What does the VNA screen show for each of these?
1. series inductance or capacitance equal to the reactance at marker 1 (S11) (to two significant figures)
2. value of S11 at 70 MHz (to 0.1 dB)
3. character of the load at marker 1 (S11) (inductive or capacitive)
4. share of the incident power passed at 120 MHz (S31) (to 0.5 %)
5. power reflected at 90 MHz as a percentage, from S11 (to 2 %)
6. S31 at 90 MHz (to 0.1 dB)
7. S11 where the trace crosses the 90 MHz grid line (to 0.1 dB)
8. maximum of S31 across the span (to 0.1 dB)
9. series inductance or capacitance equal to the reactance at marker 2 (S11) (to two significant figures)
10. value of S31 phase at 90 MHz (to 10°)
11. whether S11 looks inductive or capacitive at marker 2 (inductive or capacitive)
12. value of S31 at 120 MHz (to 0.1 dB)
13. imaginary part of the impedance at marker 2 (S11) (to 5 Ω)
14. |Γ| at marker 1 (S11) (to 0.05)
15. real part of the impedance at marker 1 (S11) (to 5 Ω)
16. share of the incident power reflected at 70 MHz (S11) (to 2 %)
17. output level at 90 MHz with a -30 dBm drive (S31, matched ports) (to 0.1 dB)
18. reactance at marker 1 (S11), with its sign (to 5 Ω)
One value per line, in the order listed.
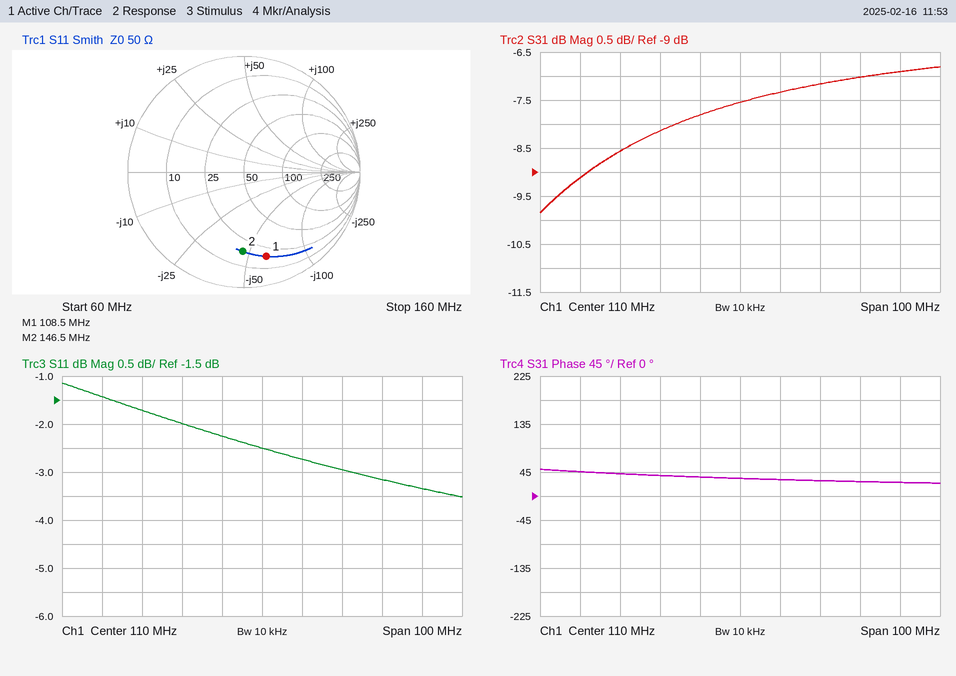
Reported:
24 pF
-1.4 dB
capacitive
18.5 %
64 %
-8.1 dB
-2.0 dB
-6.8 dB
24 pF
40°
capacitive
-7.3 dB
-45 Ω
0.75
20 Ω
72 %
-38.1 dBm
-60 Ω
